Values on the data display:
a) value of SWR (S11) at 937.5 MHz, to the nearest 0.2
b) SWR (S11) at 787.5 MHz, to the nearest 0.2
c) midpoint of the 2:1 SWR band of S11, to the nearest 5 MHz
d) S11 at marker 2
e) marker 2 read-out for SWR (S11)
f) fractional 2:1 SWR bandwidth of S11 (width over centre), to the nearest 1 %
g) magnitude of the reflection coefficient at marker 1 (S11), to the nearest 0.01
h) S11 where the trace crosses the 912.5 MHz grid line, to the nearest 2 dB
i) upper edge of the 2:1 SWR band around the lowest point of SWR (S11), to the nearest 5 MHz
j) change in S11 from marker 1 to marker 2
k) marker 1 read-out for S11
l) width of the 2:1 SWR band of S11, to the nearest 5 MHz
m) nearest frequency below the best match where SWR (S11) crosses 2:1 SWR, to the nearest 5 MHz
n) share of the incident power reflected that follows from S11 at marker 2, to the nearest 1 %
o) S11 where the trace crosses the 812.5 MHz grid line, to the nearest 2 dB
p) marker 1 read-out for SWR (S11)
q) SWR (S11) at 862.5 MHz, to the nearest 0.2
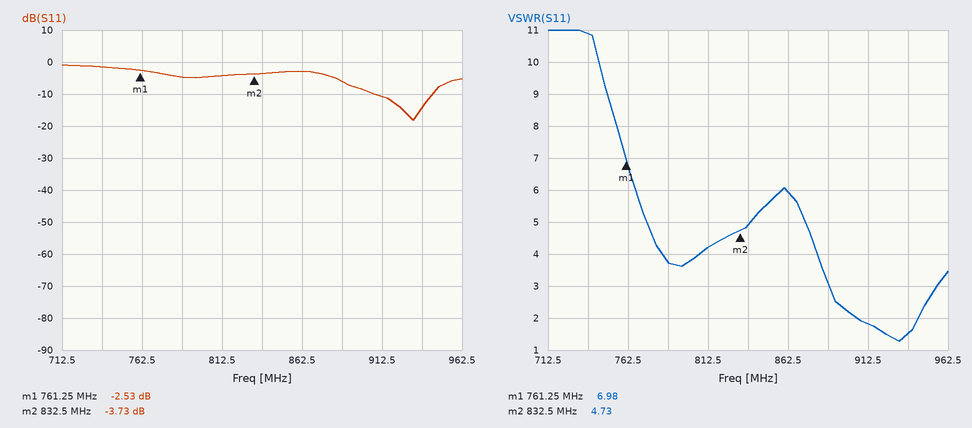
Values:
1.6
3.8
925 MHz
-3.73 dB
4.73
4 %
0.75
-10 dB
945 MHz
-1.20 dB
-2.53 dB
40 MHz
905 MHz
42 %
-4 dB
6.98
6.0
